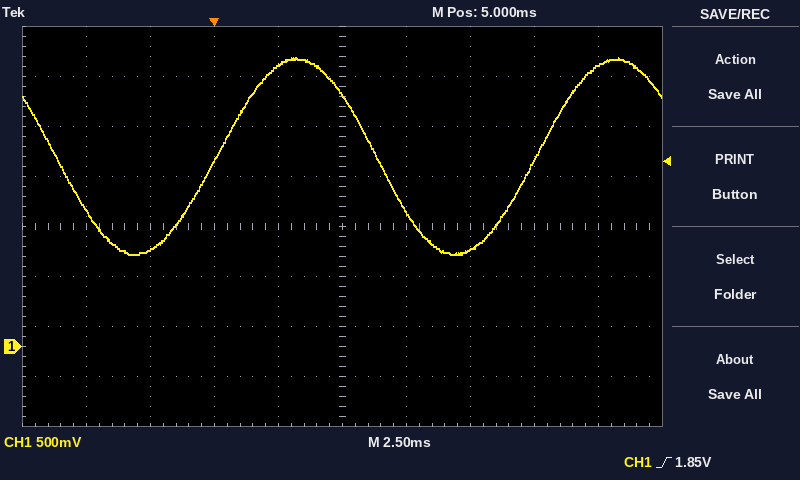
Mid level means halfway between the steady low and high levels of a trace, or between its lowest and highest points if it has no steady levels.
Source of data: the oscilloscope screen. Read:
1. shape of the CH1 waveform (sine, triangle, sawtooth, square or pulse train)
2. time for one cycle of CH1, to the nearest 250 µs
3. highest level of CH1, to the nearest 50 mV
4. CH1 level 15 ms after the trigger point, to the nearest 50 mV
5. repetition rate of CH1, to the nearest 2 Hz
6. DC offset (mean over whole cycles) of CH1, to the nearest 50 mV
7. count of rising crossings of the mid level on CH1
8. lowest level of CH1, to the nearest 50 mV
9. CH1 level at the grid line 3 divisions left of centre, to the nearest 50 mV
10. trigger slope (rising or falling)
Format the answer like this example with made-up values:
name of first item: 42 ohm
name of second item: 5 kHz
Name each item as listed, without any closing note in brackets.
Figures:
shape of the CH1 waveform: sine
time for one cycle of CH1, to the nearest 250 µs: 12.50 ms
highest level of CH1, to the nearest 50 mV: 2.90 V
CH1 level 15 ms after the trigger point, to the nearest 50 mV: 2.80 V
repetition rate of CH1, to the nearest 2 Hz: 80 Hz
DC offset (mean over whole cycles) of CH1, to the nearest 50 mV: 1.90 V
count of rising crossings of the mid level on CH1: 2
lowest level of CH1, to the nearest 50 mV: 900 mV
CH1 level at the grid line 3 divisions left of centre, to the nearest 50 mV: 950 mV
trigger slope: rising
